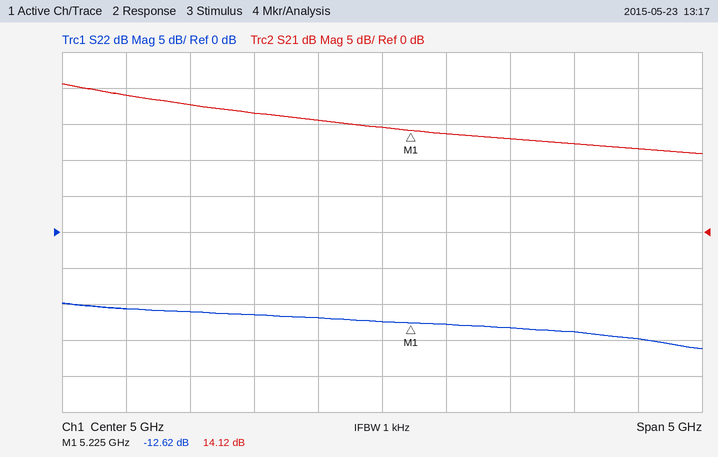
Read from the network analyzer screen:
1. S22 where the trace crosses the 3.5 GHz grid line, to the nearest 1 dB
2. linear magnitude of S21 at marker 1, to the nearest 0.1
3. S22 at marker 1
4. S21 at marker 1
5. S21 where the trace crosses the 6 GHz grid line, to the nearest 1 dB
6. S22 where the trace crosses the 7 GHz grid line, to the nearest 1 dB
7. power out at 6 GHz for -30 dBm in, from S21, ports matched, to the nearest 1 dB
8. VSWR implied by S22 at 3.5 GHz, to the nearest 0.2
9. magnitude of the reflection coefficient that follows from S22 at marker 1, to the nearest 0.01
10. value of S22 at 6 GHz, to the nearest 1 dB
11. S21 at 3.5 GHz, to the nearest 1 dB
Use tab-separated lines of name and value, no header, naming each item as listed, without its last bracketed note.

S22 where the trace crosses the 3.5 GHz grid line, to the nearest 1 dB	-11 dB
linear magnitude of S21 at marker 1, to the nearest 0.1	5.1
S22 at marker 1	-12.62 dB
S21 at marker 1	14.12 dB
S21 where the trace crosses the 6 GHz grid line, to the nearest 1 dB	13 dB
S22 where the trace crosses the 7 GHz grid line, to the nearest 1 dB	-15 dB
power out at 6 GHz for -30 dBm in, from S21, ports matched, to the nearest 1 dB	-17 dBm
VSWR implied by S22 at 3.5 GHz, to the nearest 0.2	1.8
magnitude of the reflection coefficient that follows from S22 at marker 1, to the nearest 0.01	0.23
value of S22 at 6 GHz, to the nearest 1 dB	-13 dB
S21 at 3.5 GHz, to the nearest 1 dB	18 dB
